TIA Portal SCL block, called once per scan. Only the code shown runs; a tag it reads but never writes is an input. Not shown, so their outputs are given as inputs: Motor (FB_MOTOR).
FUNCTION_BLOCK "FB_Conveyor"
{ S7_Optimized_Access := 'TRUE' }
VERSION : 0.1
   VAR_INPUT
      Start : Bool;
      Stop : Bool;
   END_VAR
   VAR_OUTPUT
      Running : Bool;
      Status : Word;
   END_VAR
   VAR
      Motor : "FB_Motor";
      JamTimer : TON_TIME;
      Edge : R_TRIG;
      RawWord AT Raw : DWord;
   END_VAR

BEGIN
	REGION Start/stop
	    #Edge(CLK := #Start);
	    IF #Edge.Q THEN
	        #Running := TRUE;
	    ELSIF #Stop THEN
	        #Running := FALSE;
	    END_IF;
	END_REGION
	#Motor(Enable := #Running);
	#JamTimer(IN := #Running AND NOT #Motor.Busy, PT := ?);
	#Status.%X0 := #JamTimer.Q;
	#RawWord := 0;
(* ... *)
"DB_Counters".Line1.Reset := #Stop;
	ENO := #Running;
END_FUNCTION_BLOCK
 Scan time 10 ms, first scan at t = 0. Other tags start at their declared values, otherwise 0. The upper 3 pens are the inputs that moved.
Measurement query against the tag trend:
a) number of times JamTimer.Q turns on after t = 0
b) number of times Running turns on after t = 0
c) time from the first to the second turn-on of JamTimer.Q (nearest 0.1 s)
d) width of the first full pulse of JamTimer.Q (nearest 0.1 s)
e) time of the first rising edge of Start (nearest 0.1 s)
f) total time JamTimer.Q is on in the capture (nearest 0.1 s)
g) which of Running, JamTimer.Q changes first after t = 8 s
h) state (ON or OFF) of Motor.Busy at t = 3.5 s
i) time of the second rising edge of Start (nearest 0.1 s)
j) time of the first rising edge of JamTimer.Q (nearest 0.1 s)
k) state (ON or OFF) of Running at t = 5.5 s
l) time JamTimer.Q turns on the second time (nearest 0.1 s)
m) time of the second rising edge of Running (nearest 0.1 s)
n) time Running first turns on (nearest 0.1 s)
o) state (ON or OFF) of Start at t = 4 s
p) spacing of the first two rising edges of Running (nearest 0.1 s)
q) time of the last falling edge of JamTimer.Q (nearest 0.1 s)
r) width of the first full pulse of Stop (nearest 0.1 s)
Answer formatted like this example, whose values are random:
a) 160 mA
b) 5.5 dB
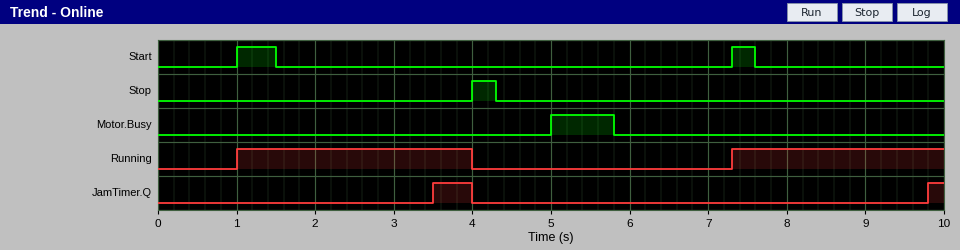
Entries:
a) 2
b) 2
c) 6.3 s
d) 0.5 s
e) 1.0 s
f) 0.7 s
g) JamTimer.Q
h) OFF
i) 7.3 s
j) 3.5 s
k) OFF
l) 9.8 s
m) 7.3 s
n) 1.0 s
o) OFF
p) 6.3 s
q) 4.0 s
r) 0.3 s
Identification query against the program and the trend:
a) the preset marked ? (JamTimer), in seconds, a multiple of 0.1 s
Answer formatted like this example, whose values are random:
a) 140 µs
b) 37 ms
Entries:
a) 2.5 s
